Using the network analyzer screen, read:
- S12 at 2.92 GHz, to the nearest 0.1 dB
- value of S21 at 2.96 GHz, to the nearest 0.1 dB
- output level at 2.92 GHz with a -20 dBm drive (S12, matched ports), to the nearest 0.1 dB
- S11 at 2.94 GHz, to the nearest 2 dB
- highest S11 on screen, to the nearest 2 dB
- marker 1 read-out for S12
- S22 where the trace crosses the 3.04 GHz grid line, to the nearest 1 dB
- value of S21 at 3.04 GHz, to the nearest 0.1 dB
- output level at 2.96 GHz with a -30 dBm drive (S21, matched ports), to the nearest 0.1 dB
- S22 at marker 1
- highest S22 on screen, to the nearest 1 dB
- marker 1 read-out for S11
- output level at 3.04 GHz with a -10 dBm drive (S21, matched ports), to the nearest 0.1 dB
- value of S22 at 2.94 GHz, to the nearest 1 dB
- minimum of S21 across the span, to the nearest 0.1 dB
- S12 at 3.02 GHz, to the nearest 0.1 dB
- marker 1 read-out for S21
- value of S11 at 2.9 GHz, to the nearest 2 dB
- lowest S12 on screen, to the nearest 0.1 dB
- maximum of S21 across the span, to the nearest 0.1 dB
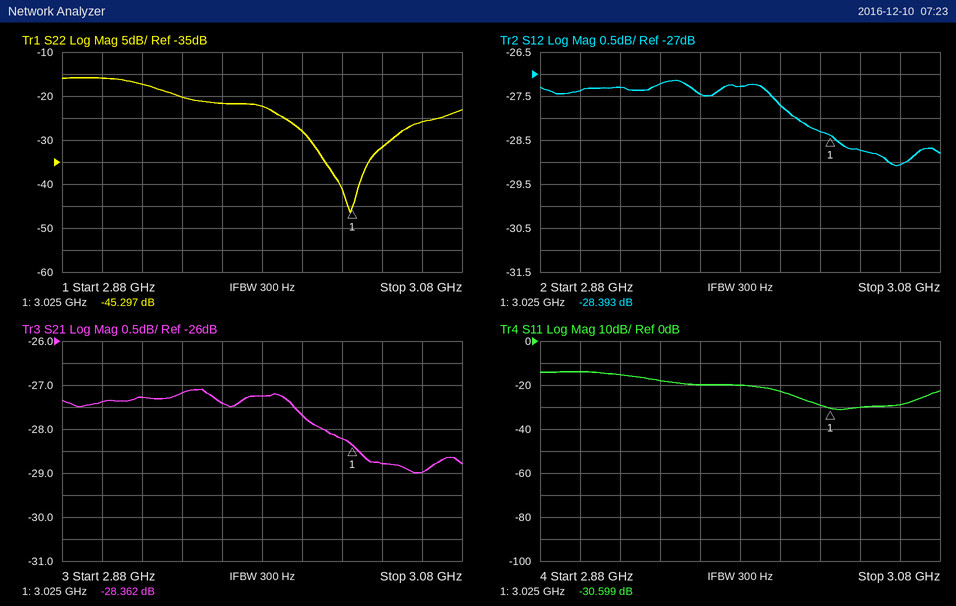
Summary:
-27.3 dB
-27.4 dB
-47.3 dBm
-18 dB
-14 dB
-28.393 dB
-32 dB
-28.8 dB
-57.4 dBm
-45.297 dB
-16 dB
-30.599 dB
-38.8 dBm
-20 dB
-29.0 dB
-28.3 dB
-28.362 dB
-14 dB
-29.1 dB
-27.1 dB
